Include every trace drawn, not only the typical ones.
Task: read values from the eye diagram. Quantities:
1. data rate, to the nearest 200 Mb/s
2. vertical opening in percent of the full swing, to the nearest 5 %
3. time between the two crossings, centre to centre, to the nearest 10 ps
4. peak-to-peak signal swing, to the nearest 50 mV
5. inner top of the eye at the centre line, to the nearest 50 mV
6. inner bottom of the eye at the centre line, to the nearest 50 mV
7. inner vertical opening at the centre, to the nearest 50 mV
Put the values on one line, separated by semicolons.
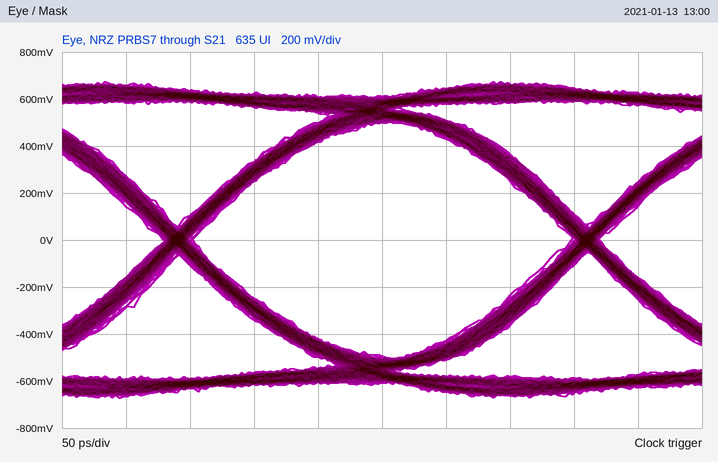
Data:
3.2 Gb/s; 75 %; 320 ps; 1.35 V; 500 mV; -500 mV; 1.00 V
